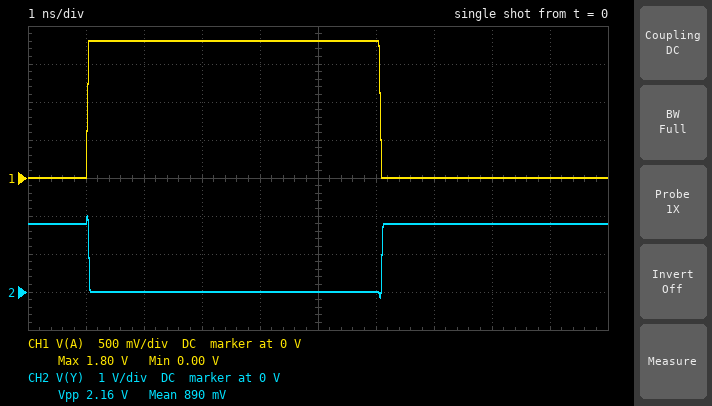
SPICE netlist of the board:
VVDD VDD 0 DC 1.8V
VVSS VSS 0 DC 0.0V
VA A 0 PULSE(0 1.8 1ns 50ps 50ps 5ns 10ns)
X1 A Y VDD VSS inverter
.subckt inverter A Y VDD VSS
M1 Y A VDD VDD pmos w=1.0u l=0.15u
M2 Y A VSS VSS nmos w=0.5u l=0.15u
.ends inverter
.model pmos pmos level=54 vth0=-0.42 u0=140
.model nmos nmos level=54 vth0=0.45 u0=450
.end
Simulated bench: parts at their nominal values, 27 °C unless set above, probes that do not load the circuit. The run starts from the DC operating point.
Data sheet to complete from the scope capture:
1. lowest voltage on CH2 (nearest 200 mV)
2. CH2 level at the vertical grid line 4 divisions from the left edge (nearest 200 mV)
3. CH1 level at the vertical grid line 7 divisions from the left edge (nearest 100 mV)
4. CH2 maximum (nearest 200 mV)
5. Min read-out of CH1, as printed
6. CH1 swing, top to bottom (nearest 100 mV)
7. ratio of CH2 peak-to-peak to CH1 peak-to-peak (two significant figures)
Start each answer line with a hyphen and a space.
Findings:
- -200 mV
- 0 V
- 0 V
- 2.0 V
- 0.00 V
- 1.8 V
- 1.2
